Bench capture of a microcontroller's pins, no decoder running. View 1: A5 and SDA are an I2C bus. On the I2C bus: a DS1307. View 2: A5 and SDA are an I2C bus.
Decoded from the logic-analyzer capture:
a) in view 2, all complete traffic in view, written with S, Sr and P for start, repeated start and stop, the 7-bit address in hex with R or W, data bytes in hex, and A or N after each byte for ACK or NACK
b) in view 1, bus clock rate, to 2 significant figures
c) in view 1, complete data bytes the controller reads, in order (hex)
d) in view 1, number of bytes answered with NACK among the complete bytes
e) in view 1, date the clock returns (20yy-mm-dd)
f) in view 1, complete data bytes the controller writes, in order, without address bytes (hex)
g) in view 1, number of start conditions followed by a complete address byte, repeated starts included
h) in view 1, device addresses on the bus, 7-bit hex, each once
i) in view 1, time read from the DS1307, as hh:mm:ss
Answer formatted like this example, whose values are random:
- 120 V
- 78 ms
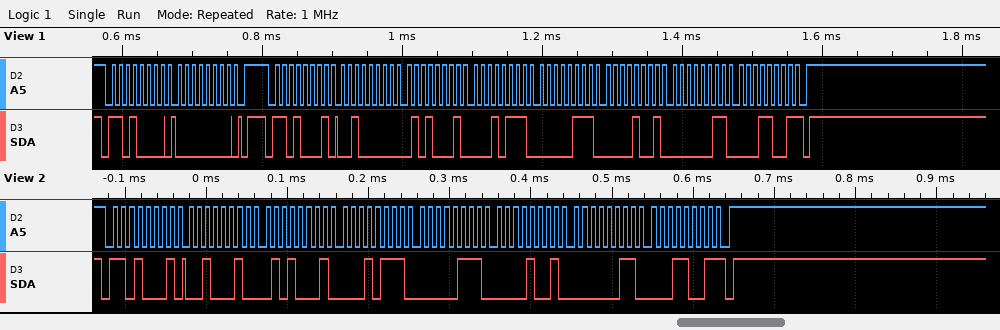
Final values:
- S 68R A 22 A 51 A 17 A 07 A 09 A 03 A 19 N P
- 100 kHz
- 20 51 17 07 09 03 19
- 1
- 2019-03-09
- 00
- 2
- 0x68
- 17:51:20
